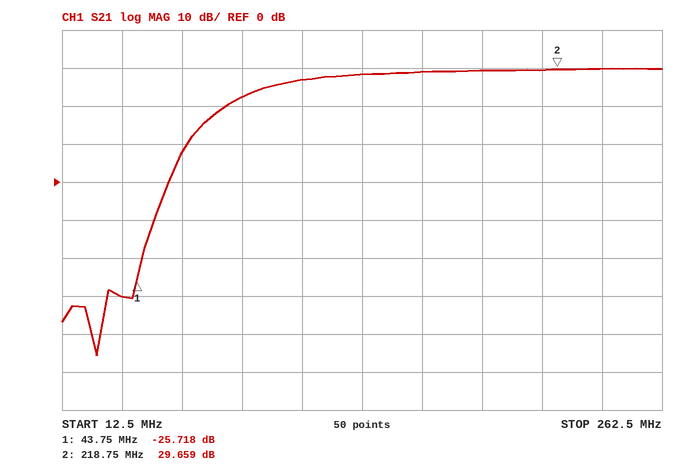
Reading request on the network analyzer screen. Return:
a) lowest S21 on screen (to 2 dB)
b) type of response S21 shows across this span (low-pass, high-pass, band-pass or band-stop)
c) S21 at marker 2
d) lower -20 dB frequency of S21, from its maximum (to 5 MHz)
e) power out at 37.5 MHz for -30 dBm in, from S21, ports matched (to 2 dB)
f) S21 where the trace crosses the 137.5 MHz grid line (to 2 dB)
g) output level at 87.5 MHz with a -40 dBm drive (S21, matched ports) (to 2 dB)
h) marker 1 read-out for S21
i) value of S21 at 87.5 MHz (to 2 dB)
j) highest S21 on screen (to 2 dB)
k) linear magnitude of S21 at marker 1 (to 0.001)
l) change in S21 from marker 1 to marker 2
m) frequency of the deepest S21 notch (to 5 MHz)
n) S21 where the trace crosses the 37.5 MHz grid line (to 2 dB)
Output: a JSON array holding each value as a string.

["-46 dB", "high-pass", "29.659 dB", "65 MHz", "-60 dBm", "28 dB", "-18 dBm", "-25.718 dB", "22 dB", "30 dB", "0.052", "55.377 dB", "25 MHz", "-30 dB"]
